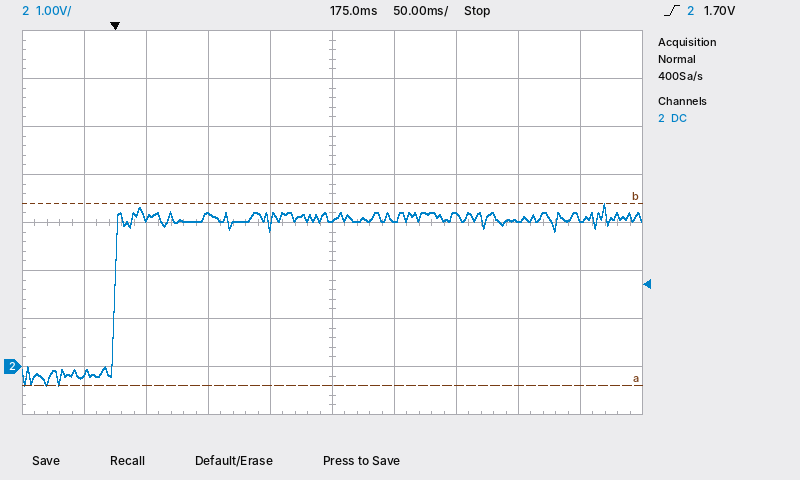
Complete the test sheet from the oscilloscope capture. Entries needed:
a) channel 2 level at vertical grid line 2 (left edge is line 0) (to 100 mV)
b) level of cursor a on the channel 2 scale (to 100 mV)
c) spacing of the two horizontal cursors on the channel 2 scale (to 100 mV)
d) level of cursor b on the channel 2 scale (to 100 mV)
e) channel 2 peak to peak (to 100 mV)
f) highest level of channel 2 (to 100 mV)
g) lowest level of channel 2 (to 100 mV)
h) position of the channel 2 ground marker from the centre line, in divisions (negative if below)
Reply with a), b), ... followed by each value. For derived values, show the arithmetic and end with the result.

a) 3.1 V
b) -400 mV
c) 3.8 V
d) 3.4 V
e) 3.4 V − (-400 mV) = 3.8 V
f) 3.4 V
g) -400 mV
h) -3.0 div
